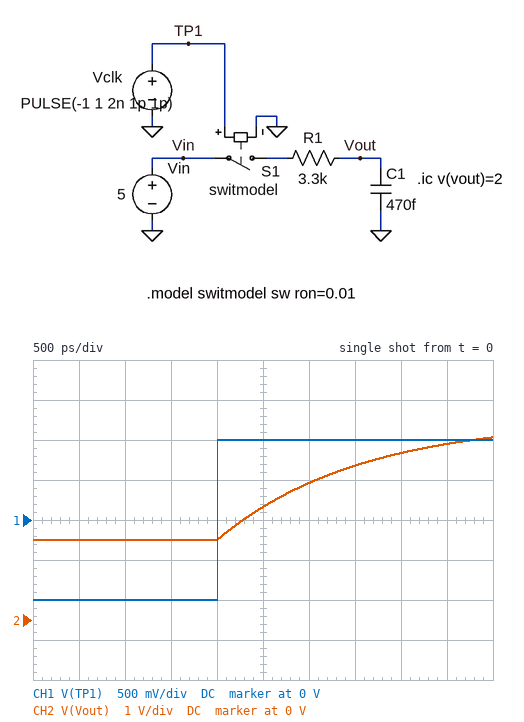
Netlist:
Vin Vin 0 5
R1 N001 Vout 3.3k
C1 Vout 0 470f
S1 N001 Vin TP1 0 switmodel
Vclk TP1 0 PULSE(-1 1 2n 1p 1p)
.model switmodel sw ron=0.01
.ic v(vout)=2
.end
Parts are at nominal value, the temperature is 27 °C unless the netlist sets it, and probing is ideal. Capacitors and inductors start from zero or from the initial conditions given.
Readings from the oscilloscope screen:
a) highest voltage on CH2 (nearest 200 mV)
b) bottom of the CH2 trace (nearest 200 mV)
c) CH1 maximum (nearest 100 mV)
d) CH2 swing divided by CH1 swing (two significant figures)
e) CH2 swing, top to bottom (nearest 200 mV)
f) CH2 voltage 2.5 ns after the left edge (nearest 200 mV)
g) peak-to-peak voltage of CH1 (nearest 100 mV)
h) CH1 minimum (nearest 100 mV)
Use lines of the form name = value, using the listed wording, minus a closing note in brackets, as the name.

highest voltage on CH2 = 4.6 V
bottom of the CH2 trace = 2.0 V
CH1 maximum = 1.0 V
CH2 swing divided by CH1 swing = 1.3
CH2 swing, top to bottom = 2.6 V
CH2 voltage 2.5 ns after the left edge = 2.8 V
peak-to-peak voltage of CH1 = 2.0 V
CH1 minimum = -1.0 V
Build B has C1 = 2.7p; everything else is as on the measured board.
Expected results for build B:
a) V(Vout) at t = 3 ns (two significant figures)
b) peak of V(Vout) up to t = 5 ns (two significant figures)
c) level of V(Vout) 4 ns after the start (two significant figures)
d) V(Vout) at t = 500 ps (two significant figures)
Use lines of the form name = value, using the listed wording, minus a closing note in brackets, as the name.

V(Vout) at t = 3 ns = 2.3 V
peak of V(Vout) up to t = 5 ns = 2.9 V
level of V(Vout) 4 ns after the start = 2.6 V
V(Vout) at t = 500 ps = 2.0 V
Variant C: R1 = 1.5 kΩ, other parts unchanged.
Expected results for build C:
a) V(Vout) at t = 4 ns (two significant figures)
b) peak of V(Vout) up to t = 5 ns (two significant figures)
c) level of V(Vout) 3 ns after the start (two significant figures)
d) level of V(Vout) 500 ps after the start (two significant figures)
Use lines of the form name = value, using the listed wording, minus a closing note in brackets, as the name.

V(Vout) at t = 4 ns = 4.8 V
peak of V(Vout) up to t = 5 ns = 5.0 V
level of V(Vout) 3 ns after the start = 4.3 V
level of V(Vout) 500 ps after the start = 2.0 V
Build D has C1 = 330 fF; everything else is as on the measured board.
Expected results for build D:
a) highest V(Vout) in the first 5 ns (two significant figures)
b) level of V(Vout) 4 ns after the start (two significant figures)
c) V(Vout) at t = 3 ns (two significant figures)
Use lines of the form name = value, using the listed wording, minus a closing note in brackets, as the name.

highest V(Vout) in the first 5 ns = 4.8 V
level of V(Vout) 4 ns after the start = 4.5 V
V(Vout) at t = 3 ns = 3.8 V
